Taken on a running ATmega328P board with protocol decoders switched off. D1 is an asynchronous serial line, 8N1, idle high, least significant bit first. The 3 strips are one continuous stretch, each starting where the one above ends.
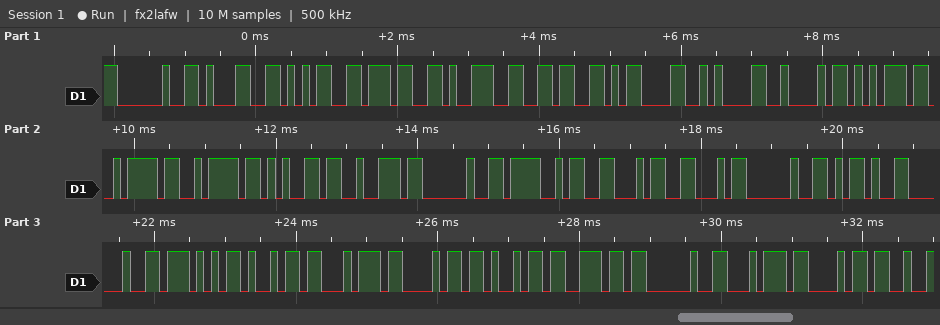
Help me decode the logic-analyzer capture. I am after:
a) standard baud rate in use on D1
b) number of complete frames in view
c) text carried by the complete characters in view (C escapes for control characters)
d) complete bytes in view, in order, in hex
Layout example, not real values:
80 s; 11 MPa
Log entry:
9600 baud; 30; " 15796\r\nBuzzer OFF - Within th"; 20 31 35 37 39 36 0D 0A 42 75 7A 7A 65 72 20 4F 46 46 20 2D 20 57 69 74 68 69 6E 20 74 68
